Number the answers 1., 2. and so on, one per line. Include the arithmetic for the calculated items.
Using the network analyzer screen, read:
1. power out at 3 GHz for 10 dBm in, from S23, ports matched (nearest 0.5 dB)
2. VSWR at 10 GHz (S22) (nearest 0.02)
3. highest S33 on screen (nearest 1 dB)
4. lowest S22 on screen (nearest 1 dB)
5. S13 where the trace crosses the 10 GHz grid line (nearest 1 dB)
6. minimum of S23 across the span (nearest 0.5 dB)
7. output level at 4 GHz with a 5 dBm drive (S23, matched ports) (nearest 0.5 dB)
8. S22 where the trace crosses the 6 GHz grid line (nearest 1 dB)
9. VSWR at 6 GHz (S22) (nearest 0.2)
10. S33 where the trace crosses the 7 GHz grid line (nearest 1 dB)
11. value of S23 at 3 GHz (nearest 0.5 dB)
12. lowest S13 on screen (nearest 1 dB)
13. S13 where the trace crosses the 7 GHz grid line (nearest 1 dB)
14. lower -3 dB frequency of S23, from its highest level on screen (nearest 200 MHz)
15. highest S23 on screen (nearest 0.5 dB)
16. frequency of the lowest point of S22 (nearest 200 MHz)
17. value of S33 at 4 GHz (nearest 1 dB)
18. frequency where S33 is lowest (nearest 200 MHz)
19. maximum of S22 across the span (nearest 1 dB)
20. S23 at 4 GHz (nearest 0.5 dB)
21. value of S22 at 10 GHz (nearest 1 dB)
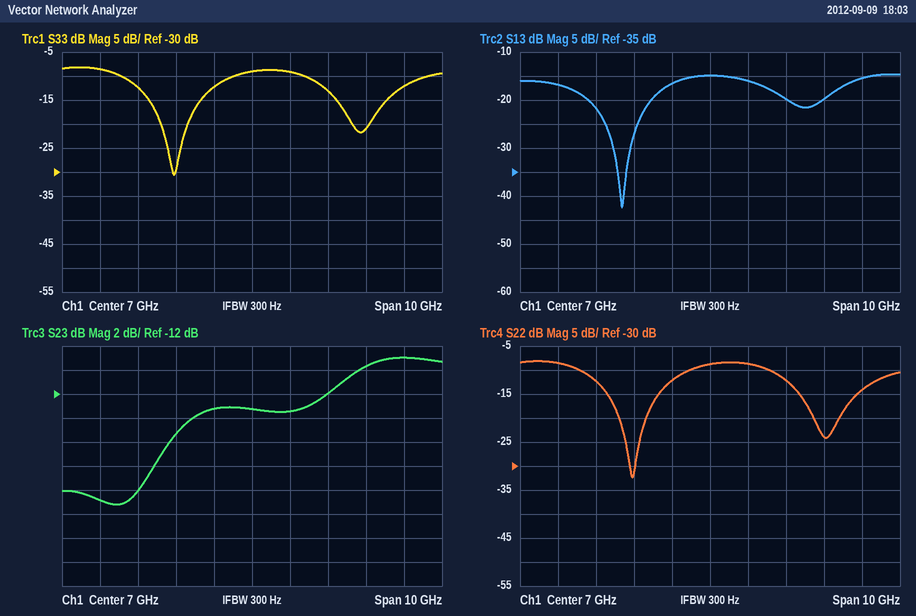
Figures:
1. 10 dBm + (-21.0 dB) = -11.0 dBm
2. |Γ| = 10^(-24/20) = 0.0631; VSWR = (1 + 0.0631)/(1 − 0.0631) ≈ 1.13, so 1.14 to the nearest 0.02
3. -8 dB
4. -32 dB
5. -20 dB
6. -21.0 dB
7. 5 dBm + (-20.0 dB) = -15.0 dBm
8. -12 dB
9. |Γ| = 10^(-12/20) = 0.2512; VSWR = (1 + 0.2512)/(1 − 0.2512) ≈ 1.67, so 1.6 to the nearest 0.2
10. -9 dB
11. -21.0 dB
12. -42 dB
13. -15 dB
14. 9.0 GHz
15. -9.0 dB
16. 5.0 GHz
17. -12 dB
18. 5.0 GHz
19. -8 dB
20. -20.0 dB
21. -24 dB
